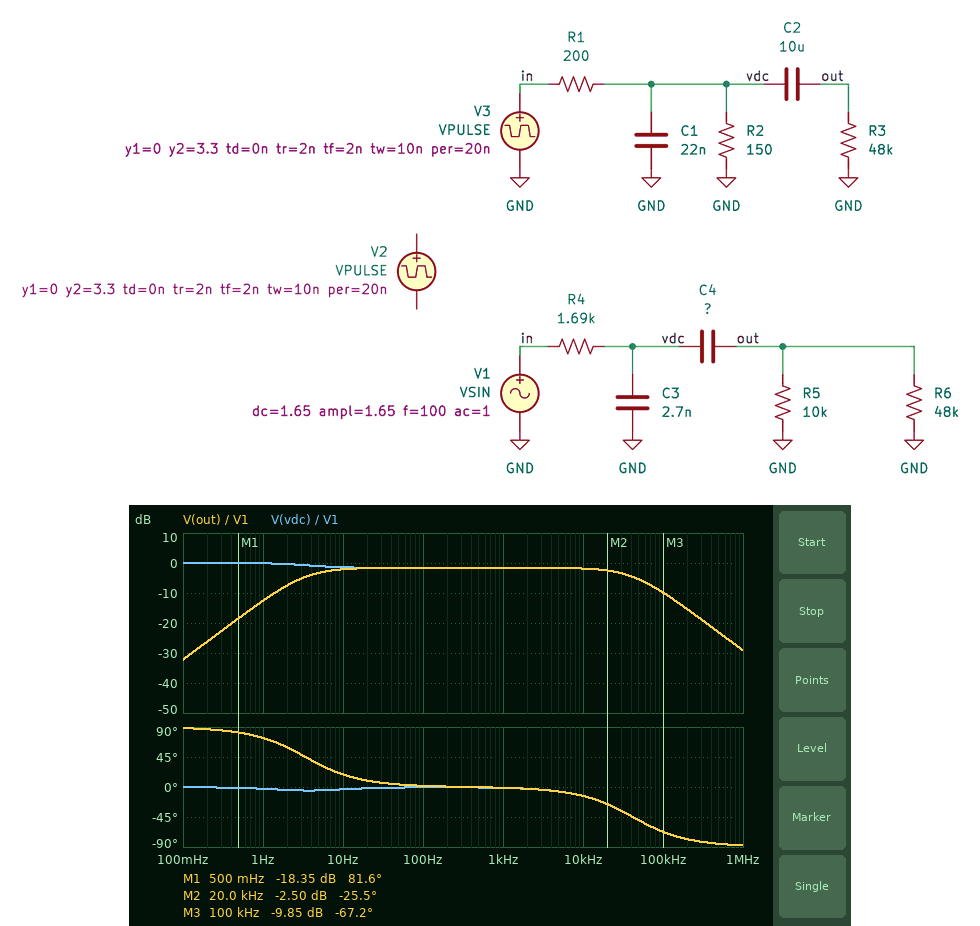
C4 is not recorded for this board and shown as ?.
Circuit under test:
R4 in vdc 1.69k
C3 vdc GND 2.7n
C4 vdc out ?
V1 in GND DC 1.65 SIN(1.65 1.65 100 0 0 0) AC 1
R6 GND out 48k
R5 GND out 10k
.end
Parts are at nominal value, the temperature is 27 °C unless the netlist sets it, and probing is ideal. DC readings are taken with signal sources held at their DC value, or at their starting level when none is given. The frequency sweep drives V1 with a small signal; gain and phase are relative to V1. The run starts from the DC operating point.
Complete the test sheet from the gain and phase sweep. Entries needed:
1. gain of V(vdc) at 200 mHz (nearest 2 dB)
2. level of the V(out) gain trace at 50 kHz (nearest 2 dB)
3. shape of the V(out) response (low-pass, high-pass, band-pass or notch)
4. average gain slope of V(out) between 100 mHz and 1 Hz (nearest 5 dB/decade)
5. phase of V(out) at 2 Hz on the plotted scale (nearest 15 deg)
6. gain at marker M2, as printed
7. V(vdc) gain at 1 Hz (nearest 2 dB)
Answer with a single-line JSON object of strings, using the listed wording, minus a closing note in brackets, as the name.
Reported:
{"gain of V(vdc) at 200 mHz": "0 dB", "level of the V(out) gain trace at 50 kHz": "-6 dB", "shape of the V(out) response": "band-pass", "average gain slope of V(out) between 100 mHz and 1 Hz": "20 dB/decade", "phase of V(out) at 2 Hz on the plotted scale": "60 deg", "gain at marker M2, as printed": "-2.50 dB", "V(vdc) gain at 1 Hz": "0 dB"}
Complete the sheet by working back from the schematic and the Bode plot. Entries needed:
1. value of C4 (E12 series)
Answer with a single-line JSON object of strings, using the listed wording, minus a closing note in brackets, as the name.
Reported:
{"value of C4": "4.7 µF"}
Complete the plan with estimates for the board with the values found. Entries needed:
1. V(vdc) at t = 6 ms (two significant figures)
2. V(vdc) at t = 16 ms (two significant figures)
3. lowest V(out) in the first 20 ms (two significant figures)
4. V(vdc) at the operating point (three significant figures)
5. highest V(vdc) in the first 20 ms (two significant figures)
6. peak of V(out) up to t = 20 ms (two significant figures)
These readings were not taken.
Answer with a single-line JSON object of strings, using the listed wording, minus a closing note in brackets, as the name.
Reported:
{"V(vdc) at t = 6 ms": "860 mV", "V(vdc) at t = 16 ms": "860 mV", "lowest V(out) in the first 20 ms": "-1.4 V", "V(vdc) at the operating point": "1.65 V", "highest V(vdc) in the first 20 ms": "3.0 V", "peak of V(out) up to t = 20 ms": "1.3 V"}
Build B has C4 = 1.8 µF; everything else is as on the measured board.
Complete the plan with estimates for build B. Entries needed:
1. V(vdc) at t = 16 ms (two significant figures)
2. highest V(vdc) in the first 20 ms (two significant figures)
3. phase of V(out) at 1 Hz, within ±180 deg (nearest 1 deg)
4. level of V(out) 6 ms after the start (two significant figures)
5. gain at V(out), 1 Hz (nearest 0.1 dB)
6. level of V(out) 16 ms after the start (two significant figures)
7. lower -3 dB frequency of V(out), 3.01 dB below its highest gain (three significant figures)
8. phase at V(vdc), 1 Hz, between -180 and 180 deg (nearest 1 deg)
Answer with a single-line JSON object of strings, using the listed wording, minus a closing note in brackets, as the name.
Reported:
{"V(vdc) at t = 16 ms": "880 mV", "highest V(vdc) in the first 20 ms": "3.0 V", "phase of V(out) at 1 Hz, within ±180 deg": "84 deg", "level of V(out) 6 ms after the start": "-980 mV", "gain at V(out), 1 Hz": "-20.6 dB", "level of V(out) 16 ms after the start": "-940 mV", "lower -3 dB frequency of V(out), 3.01 dB below its highest gain": "8.87 Hz", "phase at V(vdc), 1 Hz, between -180 and 180 deg": "-1 deg"}
